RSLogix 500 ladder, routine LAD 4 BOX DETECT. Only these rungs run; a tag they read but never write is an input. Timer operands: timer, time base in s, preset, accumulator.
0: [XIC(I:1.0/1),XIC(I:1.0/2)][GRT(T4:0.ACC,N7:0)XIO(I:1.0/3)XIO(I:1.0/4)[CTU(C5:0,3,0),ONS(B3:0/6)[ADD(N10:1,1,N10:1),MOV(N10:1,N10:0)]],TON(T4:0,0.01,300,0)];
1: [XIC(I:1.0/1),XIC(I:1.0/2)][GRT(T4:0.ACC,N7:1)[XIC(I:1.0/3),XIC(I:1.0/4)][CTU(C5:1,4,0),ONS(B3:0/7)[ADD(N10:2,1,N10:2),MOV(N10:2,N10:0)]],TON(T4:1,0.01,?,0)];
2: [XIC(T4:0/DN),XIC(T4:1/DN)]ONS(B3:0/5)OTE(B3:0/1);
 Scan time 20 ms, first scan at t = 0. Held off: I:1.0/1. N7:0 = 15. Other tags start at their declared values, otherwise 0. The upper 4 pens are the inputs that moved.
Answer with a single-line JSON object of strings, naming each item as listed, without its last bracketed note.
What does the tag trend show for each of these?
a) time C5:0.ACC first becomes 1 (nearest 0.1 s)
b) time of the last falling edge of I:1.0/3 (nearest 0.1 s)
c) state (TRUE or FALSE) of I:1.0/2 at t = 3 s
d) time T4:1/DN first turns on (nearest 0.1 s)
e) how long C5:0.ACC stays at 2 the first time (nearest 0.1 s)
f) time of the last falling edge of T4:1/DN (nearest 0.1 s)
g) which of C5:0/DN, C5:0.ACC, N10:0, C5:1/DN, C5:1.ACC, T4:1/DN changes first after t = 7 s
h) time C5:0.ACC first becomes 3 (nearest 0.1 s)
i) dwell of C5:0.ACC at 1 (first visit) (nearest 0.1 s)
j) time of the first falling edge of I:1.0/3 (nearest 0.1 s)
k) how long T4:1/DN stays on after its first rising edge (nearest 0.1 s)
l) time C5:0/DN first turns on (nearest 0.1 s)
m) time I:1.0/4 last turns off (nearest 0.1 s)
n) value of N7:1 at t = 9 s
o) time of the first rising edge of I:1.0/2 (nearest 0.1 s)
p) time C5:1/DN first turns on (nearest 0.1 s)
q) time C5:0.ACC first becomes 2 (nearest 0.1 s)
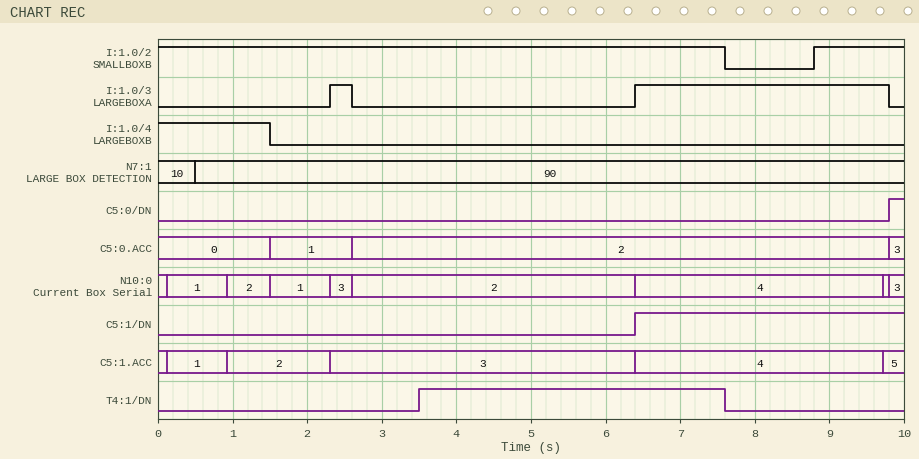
{"time C5:0.ACC first becomes 1": "1.5 s", "time of the last falling edge of I:1.0/3": "9.8 s", "state (TRUE or FALSE) of I:1.0/2 at t = 3 s": "TRUE", "time T4:1/DN first turns on": "3.5 s", "how long C5:0.ACC stays at 2 the first time": "7.2 s", "time of the last falling edge of T4:1/DN": "7.6 s", "which of C5:0/DN, C5:0.ACC, N10:0, C5:1/DN, C5:1.ACC, T4:1/DN changes first after t = 7 s": "T4:1/DN", "time C5:0.ACC first becomes 3": "9.8 s", "dwell of C5:0.ACC at 1 (first visit)": "1.1 s", "time of the first falling edge of I:1.0/3": "2.6 s", "how long T4:1/DN stays on after its first rising edge": "4.1 s", "time C5:0/DN first turns on": "9.8 s", "time I:1.0/4 last turns off": "1.5 s", "value of N7:1 at t = 9 s": "90", "time of the first rising edge of I:1.0/2": "8.8 s", "time C5:1/DN first turns on": "6.4 s", "time C5:0.ACC first becomes 2": "2.6 s"}
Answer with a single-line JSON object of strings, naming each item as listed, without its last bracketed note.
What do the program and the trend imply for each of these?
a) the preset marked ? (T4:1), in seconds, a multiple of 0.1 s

{"the preset marked ? (T4:1), in seconds, a multiple of 0.1 s": "3.5 s"}
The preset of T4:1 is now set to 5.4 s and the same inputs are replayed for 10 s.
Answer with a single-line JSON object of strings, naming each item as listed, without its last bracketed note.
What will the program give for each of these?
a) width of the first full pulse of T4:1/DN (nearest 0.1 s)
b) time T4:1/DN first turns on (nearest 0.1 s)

{"width of the first full pulse of T4:1/DN": "2.2 s", "time T4:1/DN first turns on": "5.4 s"}
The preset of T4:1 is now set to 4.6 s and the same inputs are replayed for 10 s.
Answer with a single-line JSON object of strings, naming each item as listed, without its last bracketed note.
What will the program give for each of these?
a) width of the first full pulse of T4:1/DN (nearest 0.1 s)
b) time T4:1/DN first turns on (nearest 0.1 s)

{"width of the first full pulse of T4:1/DN": "3.0 s", "time T4:1/DN first turns on": "4.6 s"}
